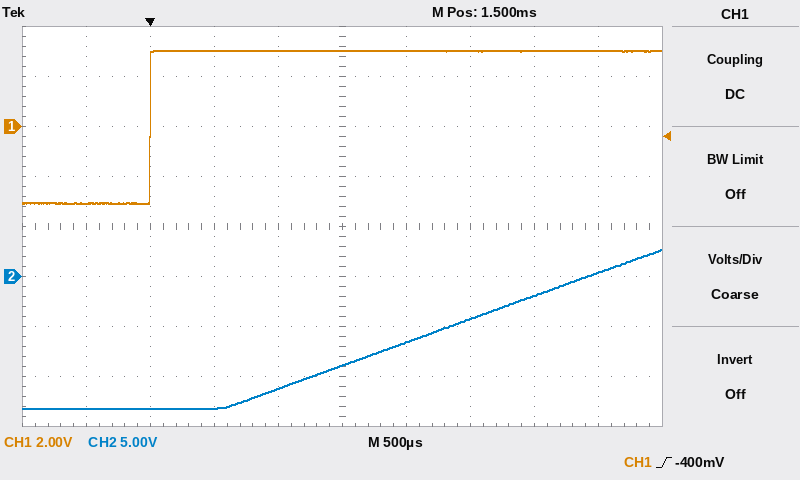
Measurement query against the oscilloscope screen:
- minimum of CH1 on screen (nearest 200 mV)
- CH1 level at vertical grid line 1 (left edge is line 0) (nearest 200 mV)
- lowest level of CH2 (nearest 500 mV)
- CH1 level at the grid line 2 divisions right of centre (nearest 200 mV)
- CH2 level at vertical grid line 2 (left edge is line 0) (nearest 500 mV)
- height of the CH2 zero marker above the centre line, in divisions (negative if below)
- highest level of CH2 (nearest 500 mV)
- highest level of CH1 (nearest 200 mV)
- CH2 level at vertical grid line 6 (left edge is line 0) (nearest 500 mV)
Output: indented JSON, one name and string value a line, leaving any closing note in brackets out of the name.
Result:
{
  "minimum of CH1 on screen": "-3.0 V",
  "CH1 level at vertical grid line 1 (left edge is line 0)": "-3.0 V",
  "lowest level of CH2": "-13.0 V",
  "CH1 level at the grid line 2 divisions right of centre": "3.0 V",
  "CH2 level at vertical grid line 2 (left edge is line 0)": "-13.0 V",
  "height of the CH2 zero marker above the centre line, in divisions": "-1.0 div",
  "highest level of CH2": "2.5 V",
  "highest level of CH1": "3.0 V",
  "CH2 level at vertical grid line 6 (left edge is line 0)": "-6.5 V"
}
